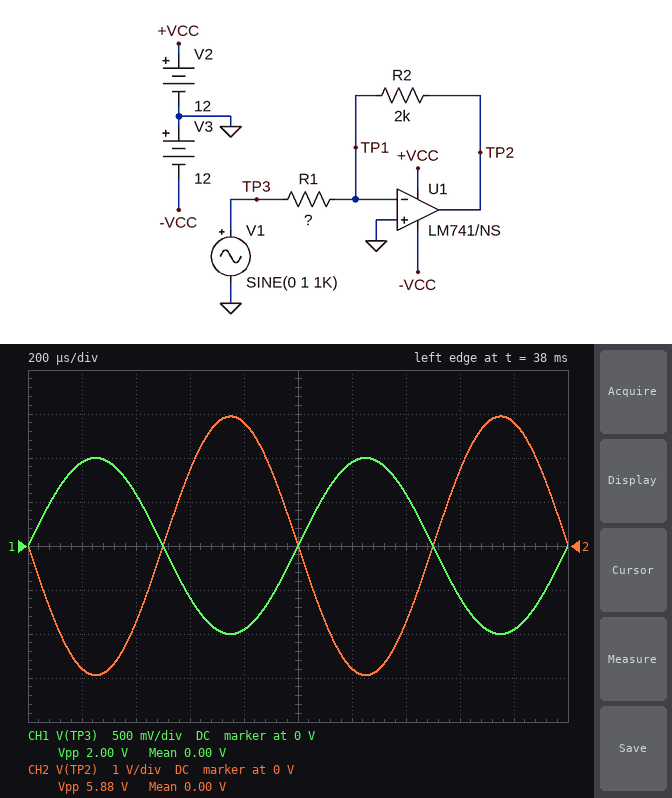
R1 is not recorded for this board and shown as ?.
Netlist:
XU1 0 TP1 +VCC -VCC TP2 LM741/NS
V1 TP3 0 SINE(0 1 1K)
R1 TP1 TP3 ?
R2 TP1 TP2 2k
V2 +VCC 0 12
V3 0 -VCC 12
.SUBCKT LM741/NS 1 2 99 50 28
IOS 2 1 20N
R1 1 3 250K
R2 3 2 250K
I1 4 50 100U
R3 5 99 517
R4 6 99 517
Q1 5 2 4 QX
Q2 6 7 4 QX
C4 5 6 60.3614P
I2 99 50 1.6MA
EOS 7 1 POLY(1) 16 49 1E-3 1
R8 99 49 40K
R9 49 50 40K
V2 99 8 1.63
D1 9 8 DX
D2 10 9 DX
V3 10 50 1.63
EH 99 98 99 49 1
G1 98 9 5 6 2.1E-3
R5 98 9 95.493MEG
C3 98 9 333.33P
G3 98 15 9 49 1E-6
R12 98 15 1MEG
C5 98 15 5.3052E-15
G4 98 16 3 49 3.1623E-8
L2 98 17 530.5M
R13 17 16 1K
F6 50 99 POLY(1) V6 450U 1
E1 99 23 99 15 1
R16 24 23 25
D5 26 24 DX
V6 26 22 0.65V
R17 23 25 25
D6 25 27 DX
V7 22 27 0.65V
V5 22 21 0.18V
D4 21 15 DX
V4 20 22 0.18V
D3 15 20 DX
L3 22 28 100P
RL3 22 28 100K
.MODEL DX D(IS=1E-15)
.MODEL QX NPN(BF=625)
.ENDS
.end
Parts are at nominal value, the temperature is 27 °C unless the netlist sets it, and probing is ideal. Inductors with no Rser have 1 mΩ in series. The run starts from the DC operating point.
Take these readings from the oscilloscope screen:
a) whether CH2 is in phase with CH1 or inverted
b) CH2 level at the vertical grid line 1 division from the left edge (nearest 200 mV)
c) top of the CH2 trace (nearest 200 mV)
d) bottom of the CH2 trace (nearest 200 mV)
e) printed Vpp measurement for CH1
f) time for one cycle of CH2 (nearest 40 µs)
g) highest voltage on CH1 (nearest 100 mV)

inverted
-2.8 V
3.0 V
-3.0 V
2.00 V
1.00 ms
1.0 V
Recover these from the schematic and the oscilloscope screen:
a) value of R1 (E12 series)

680 Ω
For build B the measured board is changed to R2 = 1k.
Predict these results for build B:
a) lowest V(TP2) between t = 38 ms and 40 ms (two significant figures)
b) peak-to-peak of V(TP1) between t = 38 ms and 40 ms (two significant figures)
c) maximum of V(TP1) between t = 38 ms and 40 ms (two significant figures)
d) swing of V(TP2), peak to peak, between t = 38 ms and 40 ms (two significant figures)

-1.5 V
3.5 mV
2.7 mV
2.9 V
